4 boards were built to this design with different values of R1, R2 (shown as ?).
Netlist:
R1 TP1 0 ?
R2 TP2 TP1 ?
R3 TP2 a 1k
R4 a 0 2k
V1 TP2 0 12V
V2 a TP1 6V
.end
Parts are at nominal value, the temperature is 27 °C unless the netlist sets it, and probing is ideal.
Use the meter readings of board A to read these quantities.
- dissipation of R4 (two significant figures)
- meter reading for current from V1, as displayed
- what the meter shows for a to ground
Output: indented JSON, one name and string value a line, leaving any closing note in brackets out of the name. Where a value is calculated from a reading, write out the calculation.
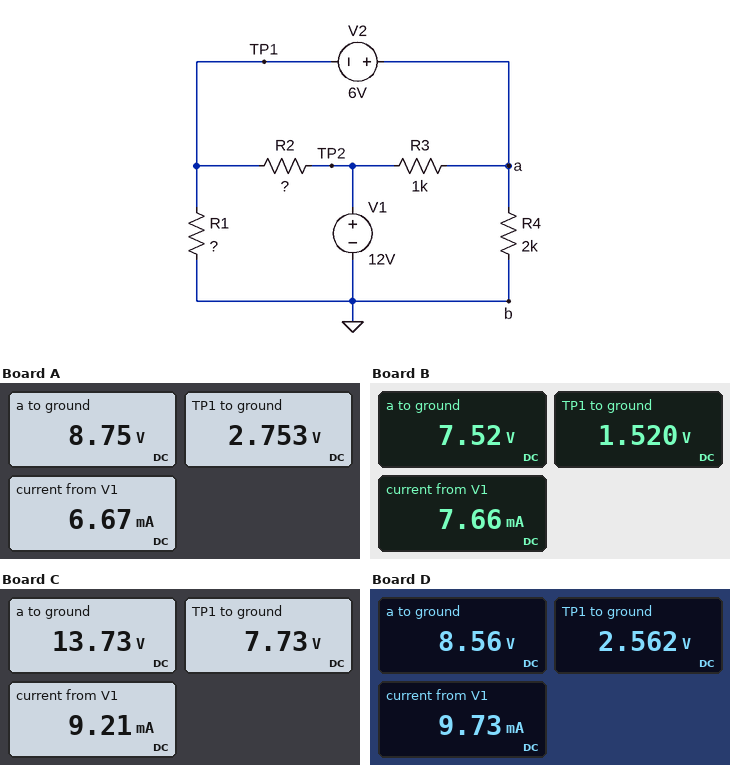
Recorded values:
{
  "dissipation of R4": "(8.75 V)^2 / 2 kΩ = 38 mW",
  "meter reading for current from V1, as displayed": "6.67 mA",
  "what the meter shows for a to ground": "8.75 V"
}
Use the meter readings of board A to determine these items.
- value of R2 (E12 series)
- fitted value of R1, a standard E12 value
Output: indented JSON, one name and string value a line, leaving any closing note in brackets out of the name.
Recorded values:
{
  "value of R2": "2.7 kΩ",
  "fitted value of R1, a standard E12 value": "1.2 kΩ"
}
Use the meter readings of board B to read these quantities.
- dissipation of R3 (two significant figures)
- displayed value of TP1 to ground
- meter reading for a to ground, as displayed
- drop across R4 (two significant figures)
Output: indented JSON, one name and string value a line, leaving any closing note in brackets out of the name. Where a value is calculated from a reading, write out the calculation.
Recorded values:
{
  "dissipation of R3": "(12 V - 7.52 V)^2 / 1 kΩ = 20 mW",
  "displayed value of TP1 to ground": "1.520 V",
  "meter reading for a to ground, as displayed": "7.52 V",
  "drop across R4": "7.52 V = 7.5 V"
}
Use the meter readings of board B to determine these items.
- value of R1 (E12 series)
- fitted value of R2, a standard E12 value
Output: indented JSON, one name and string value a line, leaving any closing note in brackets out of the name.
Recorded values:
{
  "value of R1": "390 Ω",
  "fitted value of R2, a standard E12 value": "3.3 kΩ"
}
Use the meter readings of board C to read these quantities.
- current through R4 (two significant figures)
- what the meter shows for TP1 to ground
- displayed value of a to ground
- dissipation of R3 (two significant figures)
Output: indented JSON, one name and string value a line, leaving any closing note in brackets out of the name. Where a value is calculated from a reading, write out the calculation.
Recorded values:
{
  "current through R4": "(13.73 V) / 2 kΩ = 6.9 mA",
  "what the meter shows for TP1 to ground": "7.73 V",
  "displayed value of a to ground": "13.73 V",
  "dissipation of R3": "(13.73 V - 12 V)^2 / 1 kΩ = 3.0 mW"
}
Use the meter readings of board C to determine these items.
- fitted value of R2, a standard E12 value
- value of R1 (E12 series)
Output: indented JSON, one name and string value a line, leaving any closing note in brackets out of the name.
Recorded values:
{
  "fitted value of R2, a standard E12 value": "390 Ω",
  "value of R1": "3.3 kΩ"
}
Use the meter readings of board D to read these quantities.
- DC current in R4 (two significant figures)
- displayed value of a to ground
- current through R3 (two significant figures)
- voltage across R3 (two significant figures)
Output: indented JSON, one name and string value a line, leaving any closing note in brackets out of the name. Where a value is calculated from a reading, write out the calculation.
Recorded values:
{
  "DC current in R4": "(8.56 V) / 2 kΩ = 4.3 mA",
  "displayed value of a to ground": "8.56 V",
  "current through R3": "(12 V - 8.56 V) / 1 kΩ = 3.4 mA",
  "voltage across R3": "12 V - 8.56 V = 3.4 V"
}
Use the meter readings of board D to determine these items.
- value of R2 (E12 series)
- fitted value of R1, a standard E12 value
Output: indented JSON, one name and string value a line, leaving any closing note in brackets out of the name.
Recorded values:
{
  "value of R2": "1.5 kΩ",
  "fitted value of R1, a standard E12 value": "470 Ω"
}
